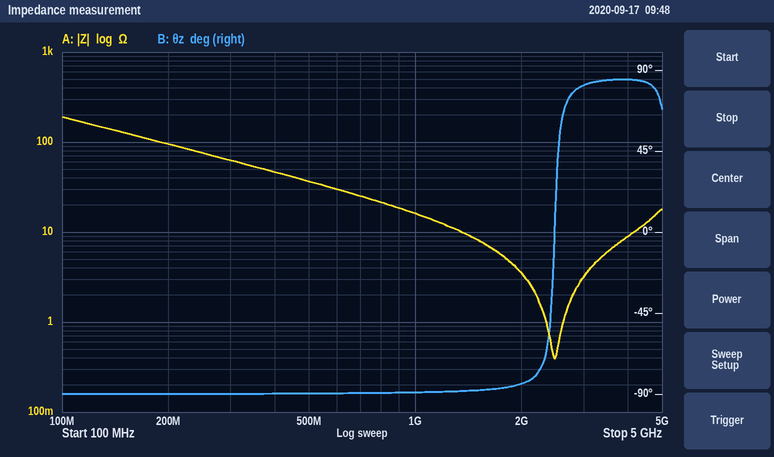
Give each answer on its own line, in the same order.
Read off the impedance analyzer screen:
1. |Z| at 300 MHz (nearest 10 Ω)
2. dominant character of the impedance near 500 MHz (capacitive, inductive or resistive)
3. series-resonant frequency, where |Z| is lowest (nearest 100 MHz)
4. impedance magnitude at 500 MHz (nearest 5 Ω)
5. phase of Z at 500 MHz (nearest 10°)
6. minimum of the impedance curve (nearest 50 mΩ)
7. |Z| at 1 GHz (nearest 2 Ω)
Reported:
60 Ω
capacitive
2.5 GHz
35 Ω
-90°
400 mΩ
16 Ω
